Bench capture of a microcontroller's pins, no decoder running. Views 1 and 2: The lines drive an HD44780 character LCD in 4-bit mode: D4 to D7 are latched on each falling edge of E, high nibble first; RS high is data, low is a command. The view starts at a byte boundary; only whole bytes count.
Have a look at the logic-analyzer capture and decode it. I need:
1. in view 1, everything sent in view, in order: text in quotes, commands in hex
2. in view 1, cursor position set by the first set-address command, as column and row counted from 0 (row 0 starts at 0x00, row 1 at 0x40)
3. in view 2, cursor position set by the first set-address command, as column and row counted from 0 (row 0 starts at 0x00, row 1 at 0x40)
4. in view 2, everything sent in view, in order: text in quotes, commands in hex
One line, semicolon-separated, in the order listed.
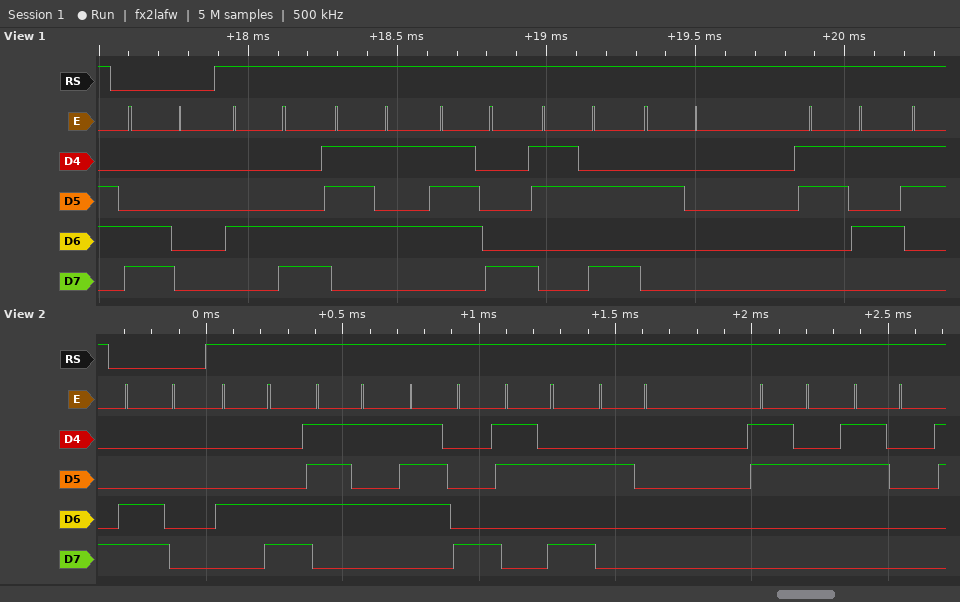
0xC0 "Lux: 5"; column 0, row 1; column 0, row 1; 0xC0 "Lux: 20"
